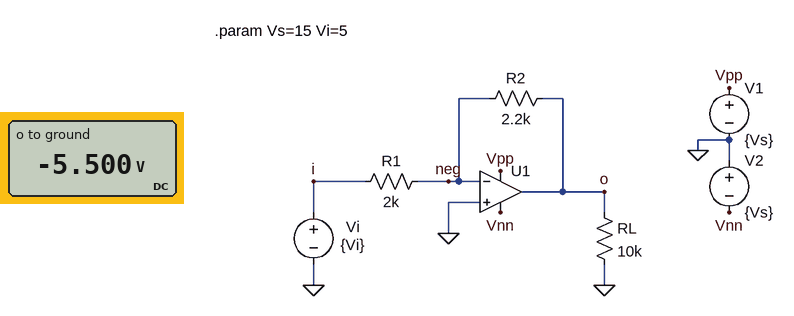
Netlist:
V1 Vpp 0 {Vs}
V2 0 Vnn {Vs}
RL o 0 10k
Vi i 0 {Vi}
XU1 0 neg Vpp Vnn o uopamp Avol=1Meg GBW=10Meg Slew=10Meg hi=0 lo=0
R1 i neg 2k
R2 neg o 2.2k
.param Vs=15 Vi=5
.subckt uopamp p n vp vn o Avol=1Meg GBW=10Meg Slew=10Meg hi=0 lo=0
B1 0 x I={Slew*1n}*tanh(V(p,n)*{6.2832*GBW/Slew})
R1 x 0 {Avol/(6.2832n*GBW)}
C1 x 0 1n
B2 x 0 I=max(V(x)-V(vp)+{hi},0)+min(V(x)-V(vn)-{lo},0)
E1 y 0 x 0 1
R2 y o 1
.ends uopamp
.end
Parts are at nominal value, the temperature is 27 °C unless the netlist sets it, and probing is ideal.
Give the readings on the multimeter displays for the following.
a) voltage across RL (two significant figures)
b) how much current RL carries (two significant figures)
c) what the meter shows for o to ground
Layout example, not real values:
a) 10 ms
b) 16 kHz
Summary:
a) 5.5 V
b) 550 µA
c) -5.500 V
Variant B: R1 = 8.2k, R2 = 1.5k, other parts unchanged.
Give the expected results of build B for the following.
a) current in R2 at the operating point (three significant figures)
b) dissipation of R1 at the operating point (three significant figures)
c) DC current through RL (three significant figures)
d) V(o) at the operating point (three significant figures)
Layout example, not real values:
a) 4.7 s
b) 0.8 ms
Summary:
a) 610 µA
b) 3.05 mW
c) 91.5 µA
d) -915 mV
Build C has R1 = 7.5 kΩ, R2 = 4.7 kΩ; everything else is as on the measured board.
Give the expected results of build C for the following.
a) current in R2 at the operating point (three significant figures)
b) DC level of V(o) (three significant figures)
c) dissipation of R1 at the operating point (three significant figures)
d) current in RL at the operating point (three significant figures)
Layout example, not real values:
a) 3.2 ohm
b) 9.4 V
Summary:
a) 667 µA
b) -3.13 V
c) 3.33 mW
d) 313 µA
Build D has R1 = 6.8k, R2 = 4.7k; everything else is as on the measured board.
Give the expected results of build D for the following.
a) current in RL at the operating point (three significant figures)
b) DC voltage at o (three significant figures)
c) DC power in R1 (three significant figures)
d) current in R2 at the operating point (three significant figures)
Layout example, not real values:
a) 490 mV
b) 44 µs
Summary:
a) 346 µA
b) -3.46 V
c) 3.68 mW
d) 735 µA
